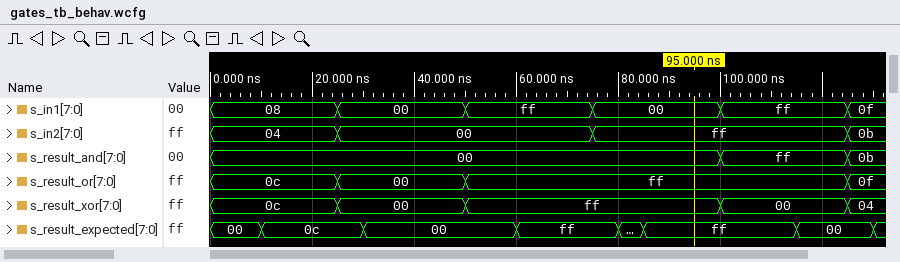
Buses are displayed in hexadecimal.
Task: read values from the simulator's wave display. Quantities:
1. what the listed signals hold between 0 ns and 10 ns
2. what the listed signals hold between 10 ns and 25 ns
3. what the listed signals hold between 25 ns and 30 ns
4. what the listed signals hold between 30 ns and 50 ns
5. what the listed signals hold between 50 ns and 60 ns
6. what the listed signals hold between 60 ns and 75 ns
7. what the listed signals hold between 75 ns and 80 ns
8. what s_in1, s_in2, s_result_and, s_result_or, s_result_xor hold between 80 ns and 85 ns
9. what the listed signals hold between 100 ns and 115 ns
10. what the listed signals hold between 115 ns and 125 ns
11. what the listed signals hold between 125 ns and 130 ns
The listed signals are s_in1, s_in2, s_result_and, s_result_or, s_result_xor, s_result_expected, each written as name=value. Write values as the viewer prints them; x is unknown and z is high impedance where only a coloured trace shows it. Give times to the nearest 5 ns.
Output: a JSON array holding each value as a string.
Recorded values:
["s_in1=08, s_in2=04, s_result_and=00, s_result_or=0c, s_result_xor=0c, s_result_expected=00", "s_in1=08, s_in2=04, s_result_and=00, s_result_or=0c, s_result_xor=0c, s_result_expected=0c", "s_in1=00, s_in2=00, s_result_and=00, s_result_or=00, s_result_xor=00, s_result_expected=0c", "s_in1=00, s_in2=00, s_result_and=00, s_result_or=00, s_result_xor=00, s_result_expected=00", "s_in1=ff, s_in2=00, s_result_and=00, s_result_or=ff, s_result_xor=ff, s_result_expected=00", "s_in1=ff, s_in2=00, s_result_and=00, s_result_or=ff, s_result_xor=ff, s_result_expected=ff", "s_in1=00, s_in2=ff, s_result_and=00, s_result_or=ff, s_result_xor=ff, s_result_expected=ff", "s_in1=00, s_in2=ff, s_result_and=00, s_result_or=ff, s_result_xor=ff", "s_in1=ff, s_in2=ff, s_result_and=ff, s_result_or=ff, s_result_xor=00, s_result_expected=ff", "s_in1=ff, s_in2=ff, s_result_and=ff, s_result_or=ff, s_result_xor=00, s_result_expected=00", "s_in1=0f, s_in2=0b, s_result_and=0b, s_result_or=0f, s_result_xor=04, s_result_expected=00"]
